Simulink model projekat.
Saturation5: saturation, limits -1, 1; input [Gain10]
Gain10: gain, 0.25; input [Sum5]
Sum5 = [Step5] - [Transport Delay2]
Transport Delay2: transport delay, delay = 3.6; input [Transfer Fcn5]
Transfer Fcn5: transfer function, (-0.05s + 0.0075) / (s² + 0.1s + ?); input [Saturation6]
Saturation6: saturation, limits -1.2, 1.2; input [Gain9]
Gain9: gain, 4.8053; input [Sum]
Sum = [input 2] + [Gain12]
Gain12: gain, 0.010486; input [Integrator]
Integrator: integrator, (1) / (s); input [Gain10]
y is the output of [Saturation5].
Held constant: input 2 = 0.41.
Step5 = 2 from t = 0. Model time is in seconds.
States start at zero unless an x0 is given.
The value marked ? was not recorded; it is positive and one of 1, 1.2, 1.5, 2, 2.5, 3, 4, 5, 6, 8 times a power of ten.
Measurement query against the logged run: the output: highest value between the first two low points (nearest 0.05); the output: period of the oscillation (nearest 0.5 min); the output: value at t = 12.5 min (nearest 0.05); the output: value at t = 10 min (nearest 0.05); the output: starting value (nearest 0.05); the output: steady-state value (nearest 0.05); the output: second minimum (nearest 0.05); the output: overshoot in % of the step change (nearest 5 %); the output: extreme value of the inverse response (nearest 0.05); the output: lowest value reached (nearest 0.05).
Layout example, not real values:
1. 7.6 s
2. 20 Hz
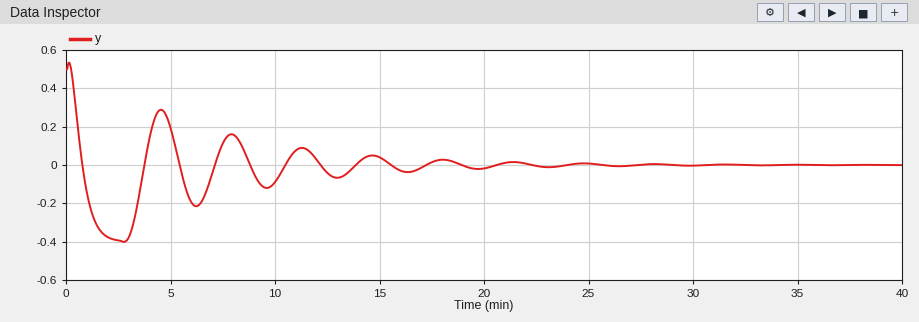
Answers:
1. 0.30
2. 3.5 min
3. -0.05
4. -0.10
5. 0.50
6. 0.00
7. -0.20
8. 80 %
9. 0.55
10. -0.40
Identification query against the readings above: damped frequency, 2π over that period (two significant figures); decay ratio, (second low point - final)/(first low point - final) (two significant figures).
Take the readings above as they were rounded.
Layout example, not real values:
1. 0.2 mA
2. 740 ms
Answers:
1. 1.8 rad/min
2. 0.50
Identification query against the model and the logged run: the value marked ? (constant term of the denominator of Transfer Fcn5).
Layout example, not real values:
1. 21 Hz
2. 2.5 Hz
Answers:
1. 0.0025
